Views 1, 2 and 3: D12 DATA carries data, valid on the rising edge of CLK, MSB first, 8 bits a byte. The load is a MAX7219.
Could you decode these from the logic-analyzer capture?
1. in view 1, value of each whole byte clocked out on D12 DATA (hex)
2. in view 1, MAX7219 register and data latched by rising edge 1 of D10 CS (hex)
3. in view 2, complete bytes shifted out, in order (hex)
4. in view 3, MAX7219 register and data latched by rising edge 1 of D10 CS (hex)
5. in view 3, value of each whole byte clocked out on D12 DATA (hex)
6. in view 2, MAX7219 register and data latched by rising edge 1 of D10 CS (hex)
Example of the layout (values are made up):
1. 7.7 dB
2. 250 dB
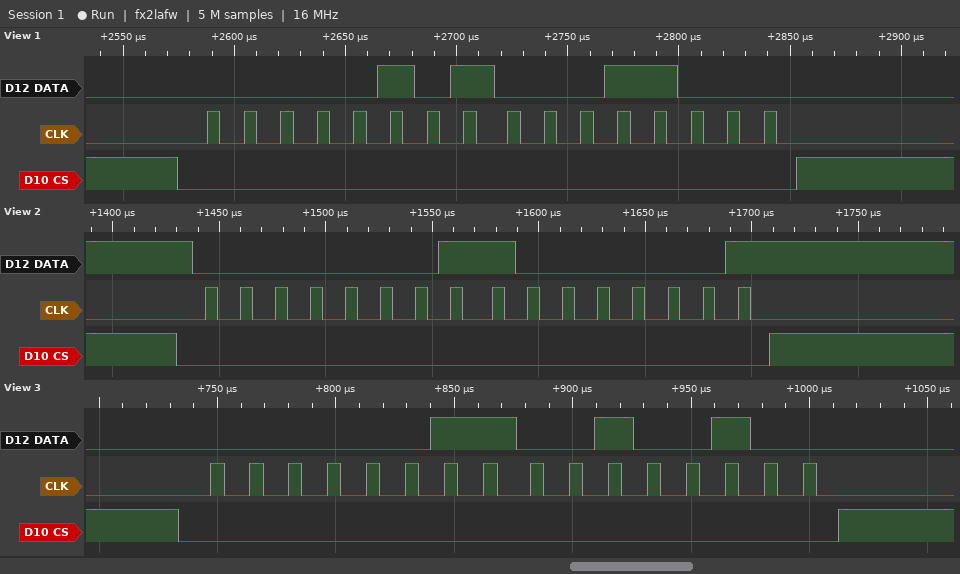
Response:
1. 05 18
2. register 0x5, data 0x18
3. 01 81
4. register 0x3, data 0x24
5. 0x03 0x24
6. register 0x1, data 0x81
